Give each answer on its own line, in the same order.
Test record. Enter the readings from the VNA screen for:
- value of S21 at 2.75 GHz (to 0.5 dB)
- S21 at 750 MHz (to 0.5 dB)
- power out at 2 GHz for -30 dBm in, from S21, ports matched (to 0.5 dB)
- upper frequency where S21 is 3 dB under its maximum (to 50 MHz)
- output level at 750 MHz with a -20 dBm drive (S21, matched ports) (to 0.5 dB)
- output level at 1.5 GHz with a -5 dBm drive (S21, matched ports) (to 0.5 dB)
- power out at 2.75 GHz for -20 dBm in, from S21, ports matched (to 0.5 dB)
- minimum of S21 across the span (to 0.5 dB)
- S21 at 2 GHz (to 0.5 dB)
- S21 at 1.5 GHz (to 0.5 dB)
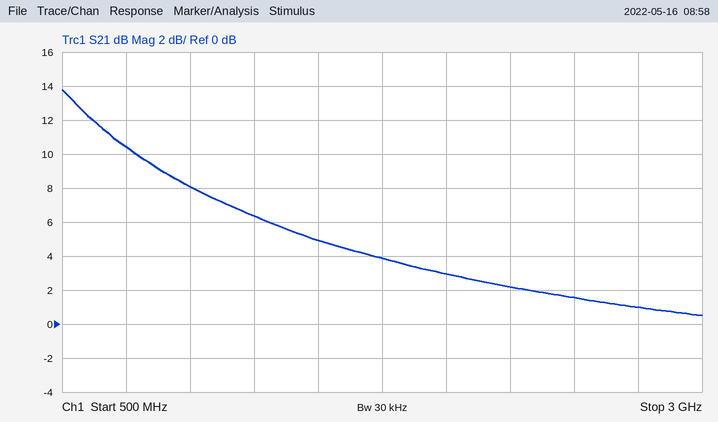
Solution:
1.0 dB
10.5 dB
-27.0 dBm
700 MHz
-9.5 dBm
0.0 dBm
-19.0 dBm
0.5 dB
3.0 dB
5.0 dB
